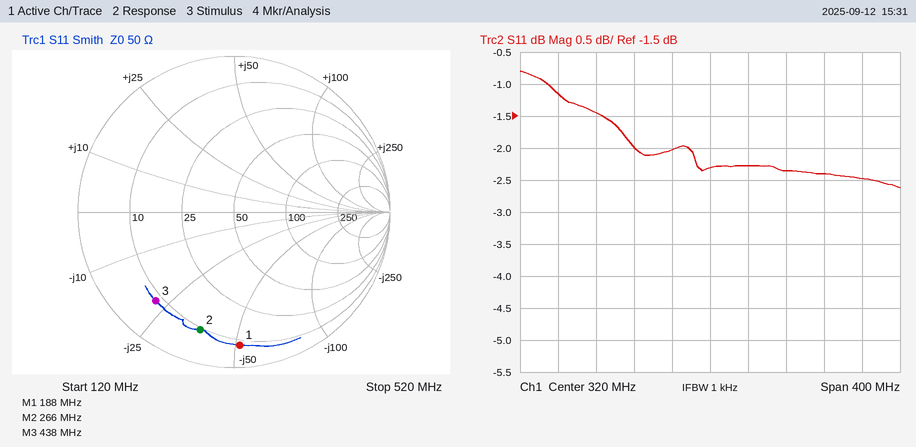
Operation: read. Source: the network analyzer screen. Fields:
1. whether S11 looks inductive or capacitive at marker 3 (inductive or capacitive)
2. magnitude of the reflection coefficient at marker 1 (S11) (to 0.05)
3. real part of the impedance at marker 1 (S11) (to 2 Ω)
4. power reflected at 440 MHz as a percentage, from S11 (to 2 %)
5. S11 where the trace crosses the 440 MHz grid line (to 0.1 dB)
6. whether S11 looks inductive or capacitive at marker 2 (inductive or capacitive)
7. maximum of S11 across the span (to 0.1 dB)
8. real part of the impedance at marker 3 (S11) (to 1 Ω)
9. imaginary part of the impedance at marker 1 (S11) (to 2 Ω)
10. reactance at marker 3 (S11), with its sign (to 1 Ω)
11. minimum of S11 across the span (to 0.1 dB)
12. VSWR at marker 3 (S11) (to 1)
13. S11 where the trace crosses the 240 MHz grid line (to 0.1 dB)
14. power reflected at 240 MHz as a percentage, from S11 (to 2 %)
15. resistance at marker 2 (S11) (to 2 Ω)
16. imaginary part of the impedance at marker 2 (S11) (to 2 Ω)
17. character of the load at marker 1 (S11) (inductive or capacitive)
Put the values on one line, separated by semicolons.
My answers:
capacitive; 0.85; 8 Ω; 58 %; -2.4 dB; capacitive; -0.8 dB; 8 Ω; -52 Ω; -22 Ω; -2.6 dB; 7; -2.0 dB; 64 %; 10 Ω; -36 Ω; capacitive
